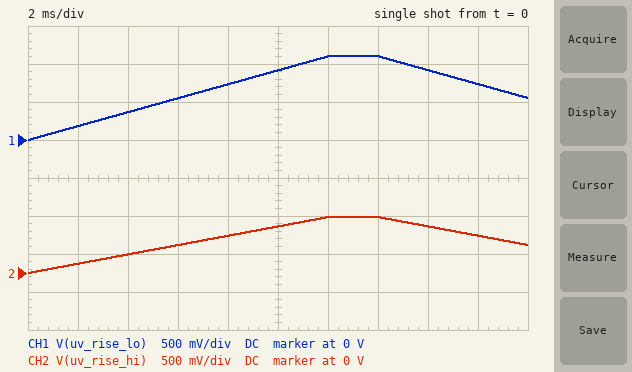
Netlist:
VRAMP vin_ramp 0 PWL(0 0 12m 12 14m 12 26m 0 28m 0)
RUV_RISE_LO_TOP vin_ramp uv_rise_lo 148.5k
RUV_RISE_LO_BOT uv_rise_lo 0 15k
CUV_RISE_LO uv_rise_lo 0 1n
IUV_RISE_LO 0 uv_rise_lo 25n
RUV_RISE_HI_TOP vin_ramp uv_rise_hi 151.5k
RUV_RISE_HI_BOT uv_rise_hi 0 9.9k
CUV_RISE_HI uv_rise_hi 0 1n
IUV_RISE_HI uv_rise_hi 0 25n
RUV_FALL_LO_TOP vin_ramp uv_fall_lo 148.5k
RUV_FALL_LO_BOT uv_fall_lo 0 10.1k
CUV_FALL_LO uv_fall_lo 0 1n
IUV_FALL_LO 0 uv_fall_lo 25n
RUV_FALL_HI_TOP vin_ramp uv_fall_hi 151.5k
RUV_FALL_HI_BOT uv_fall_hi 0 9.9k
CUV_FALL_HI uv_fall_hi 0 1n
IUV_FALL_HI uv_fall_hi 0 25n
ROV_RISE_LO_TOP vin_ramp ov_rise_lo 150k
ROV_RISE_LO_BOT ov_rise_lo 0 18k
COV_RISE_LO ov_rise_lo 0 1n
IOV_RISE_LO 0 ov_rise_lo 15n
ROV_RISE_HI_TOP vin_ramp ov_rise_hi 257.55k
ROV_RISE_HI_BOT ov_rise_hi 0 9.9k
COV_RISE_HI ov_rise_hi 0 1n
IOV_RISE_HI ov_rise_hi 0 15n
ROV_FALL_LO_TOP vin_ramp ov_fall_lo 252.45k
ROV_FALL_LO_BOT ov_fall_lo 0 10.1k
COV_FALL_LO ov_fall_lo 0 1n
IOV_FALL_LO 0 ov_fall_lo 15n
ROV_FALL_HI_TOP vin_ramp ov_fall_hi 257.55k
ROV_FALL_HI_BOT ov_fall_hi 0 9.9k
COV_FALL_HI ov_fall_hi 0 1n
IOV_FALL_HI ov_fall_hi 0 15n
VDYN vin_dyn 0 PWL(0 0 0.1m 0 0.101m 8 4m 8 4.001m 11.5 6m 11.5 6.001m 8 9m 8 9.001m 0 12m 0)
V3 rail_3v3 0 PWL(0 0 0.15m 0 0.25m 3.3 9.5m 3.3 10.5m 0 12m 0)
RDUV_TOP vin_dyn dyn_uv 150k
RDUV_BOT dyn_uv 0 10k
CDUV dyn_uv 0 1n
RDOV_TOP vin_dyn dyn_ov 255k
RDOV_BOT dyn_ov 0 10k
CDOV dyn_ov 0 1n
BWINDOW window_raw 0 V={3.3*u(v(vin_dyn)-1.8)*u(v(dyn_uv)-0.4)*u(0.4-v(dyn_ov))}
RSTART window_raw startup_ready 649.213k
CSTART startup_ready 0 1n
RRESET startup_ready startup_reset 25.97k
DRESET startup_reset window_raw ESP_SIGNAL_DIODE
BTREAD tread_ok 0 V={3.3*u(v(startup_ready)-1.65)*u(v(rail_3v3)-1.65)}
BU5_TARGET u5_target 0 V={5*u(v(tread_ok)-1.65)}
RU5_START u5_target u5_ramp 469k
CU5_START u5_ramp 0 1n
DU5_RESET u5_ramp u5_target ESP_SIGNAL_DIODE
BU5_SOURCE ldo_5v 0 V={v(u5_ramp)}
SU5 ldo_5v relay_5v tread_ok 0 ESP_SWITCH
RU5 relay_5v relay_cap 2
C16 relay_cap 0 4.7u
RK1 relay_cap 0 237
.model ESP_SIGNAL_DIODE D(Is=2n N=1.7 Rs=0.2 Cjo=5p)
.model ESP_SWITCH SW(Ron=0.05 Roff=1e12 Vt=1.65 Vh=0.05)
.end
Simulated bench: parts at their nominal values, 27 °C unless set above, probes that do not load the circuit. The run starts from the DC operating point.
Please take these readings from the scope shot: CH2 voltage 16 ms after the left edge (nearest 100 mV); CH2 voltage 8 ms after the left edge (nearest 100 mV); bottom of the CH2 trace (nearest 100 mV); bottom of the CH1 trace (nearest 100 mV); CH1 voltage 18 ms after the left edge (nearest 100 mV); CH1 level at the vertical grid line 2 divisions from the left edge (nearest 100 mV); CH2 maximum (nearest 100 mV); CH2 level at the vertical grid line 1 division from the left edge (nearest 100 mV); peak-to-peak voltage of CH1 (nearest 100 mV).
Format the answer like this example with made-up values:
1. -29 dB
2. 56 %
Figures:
1. 600 mV
2. 500 mV
3. 0 V
4. 0 V
5. 700 mV
6. 400 mV
7. 700 mV
8. 100 mV
9. 1.1 V
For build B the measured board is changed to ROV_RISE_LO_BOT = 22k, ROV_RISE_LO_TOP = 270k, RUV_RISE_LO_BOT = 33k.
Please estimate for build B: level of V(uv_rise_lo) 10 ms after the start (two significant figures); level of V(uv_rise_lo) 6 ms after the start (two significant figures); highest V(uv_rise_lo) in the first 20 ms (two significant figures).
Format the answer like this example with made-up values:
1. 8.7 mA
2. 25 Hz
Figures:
1. 1.8 V
2. 1.1 V
3. 2.2 V
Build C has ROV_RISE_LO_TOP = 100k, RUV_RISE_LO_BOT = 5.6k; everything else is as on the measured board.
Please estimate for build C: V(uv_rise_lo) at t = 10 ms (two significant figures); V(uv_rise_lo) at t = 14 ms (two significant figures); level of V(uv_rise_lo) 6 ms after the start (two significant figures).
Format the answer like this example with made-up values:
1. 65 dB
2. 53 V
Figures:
1. 360 mV
2. 440 mV
3. 220 mV
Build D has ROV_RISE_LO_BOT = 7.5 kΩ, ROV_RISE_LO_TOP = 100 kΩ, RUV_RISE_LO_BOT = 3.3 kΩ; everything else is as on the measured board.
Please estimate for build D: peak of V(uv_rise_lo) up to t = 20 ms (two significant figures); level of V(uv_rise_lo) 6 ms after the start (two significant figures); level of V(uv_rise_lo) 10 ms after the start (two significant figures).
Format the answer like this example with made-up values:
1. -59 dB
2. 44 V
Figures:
1. 260 mV
2. 130 mV
3. 220 mV
